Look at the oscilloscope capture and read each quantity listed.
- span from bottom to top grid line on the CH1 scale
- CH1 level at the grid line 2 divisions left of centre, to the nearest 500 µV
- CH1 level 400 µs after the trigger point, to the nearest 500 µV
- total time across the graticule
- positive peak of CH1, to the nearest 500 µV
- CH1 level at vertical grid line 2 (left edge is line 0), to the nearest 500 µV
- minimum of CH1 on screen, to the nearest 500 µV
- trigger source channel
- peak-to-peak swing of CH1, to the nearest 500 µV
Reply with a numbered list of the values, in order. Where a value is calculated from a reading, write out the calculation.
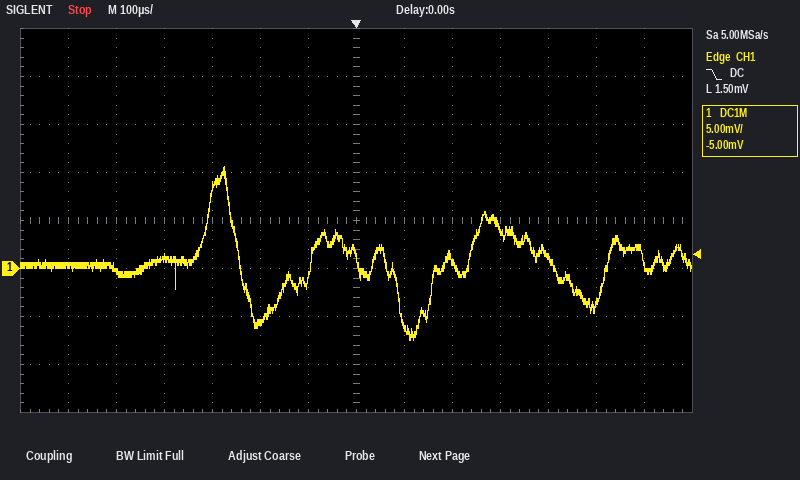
1. 40 mV
2. -5.5 mV
3. 1.0 mV
4. 1.4 ms
5. 10.5 mV
6. -500 µV
7. -7.5 mV
8. CH1
9. 10.5 mV − (-7.5 mV) = 18.0 mV
